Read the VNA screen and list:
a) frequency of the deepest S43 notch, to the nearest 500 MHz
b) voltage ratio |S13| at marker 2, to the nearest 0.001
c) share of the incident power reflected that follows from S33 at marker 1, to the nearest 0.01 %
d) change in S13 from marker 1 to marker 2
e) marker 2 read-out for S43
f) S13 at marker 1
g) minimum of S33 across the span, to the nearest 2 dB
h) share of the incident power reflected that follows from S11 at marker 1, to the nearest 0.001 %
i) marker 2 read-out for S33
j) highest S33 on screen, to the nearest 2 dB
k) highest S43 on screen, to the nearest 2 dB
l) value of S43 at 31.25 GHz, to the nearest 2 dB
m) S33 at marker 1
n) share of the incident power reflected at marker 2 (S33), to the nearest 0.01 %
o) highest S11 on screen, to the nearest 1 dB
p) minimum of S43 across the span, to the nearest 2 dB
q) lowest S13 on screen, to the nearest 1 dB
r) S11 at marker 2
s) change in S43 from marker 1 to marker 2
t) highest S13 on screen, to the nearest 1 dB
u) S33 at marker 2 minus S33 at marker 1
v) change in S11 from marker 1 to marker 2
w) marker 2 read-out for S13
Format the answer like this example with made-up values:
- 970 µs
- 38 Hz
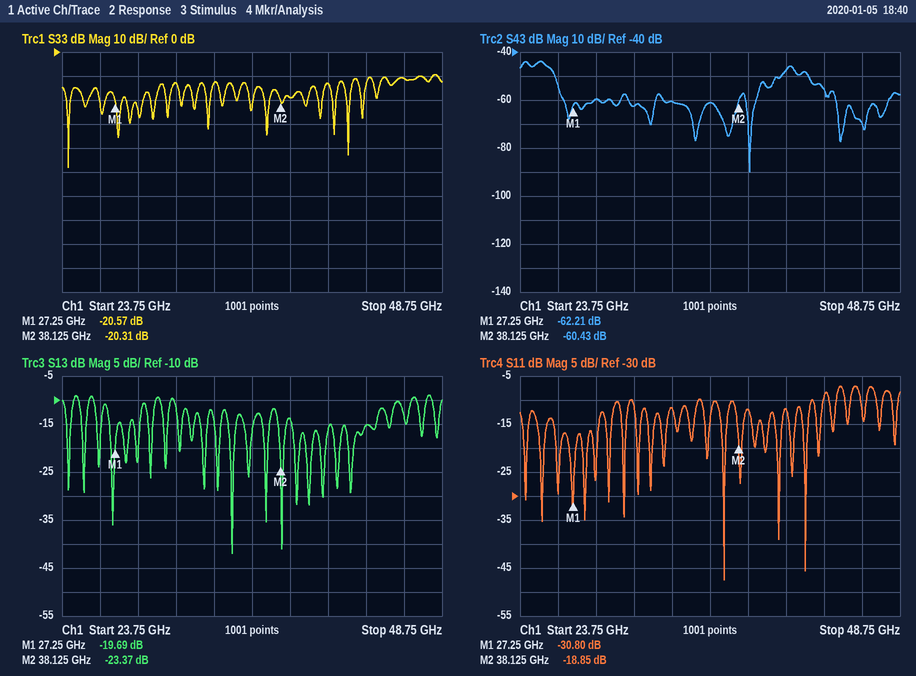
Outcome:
- 39.0 GHz
- 0.068
- 0.88 %
- -3.68 dB
- -60.43 dB
- -19.69 dB
- -48 dB
- 0.083 %
- -20.31 dB
- -10 dB
- -44 dB
- -62 dB
- -20.57 dB
- 0.93 %
- -7 dB
- -90 dB
- -42 dB
- -18.85 dB
- 1.78 dB
- -9 dB
- 0.26 dB
- 11.95 dB
- -23.37 dB
